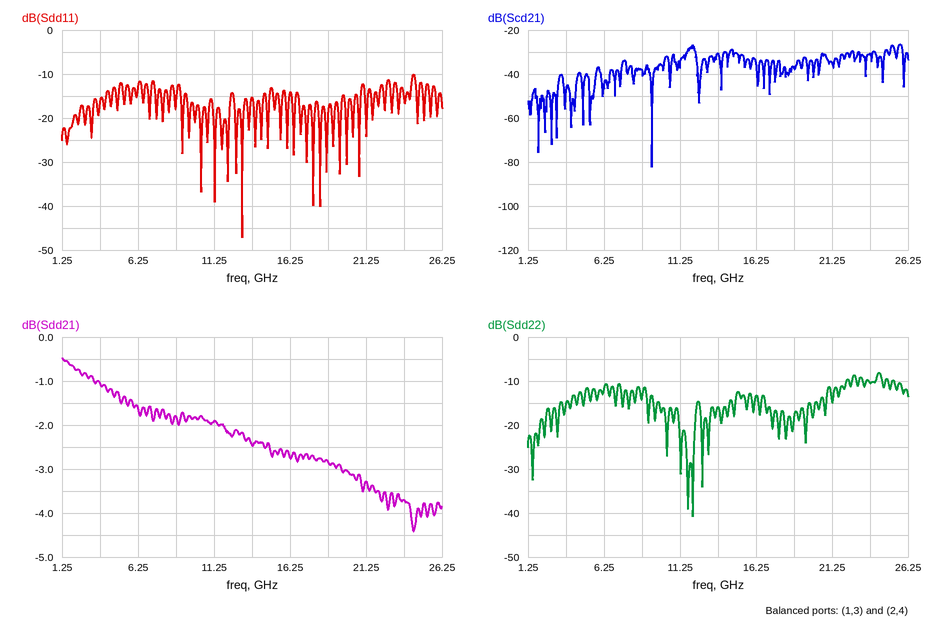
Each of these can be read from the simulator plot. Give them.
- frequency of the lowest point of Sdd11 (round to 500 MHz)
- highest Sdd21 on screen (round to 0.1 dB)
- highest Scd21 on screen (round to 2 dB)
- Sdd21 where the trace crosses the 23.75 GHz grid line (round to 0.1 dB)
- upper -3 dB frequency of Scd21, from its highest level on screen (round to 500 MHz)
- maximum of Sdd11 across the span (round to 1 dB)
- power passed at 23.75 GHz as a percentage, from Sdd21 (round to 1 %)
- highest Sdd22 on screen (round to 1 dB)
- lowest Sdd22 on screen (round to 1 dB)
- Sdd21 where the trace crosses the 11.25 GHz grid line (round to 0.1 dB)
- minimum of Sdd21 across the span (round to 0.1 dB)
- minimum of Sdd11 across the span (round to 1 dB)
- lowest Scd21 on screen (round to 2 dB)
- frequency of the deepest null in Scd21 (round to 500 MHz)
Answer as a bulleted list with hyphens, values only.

- 13.0 GHz
- -0.5 dB
- -26 dB
- -3.7 dB
- 26.0 GHz
- -10 dB
- 43 %
- -8 dB
- -41 dB
- -1.9 dB
- -4.4 dB
- -47 dB
- -82 dB
- 9.5 GHz
